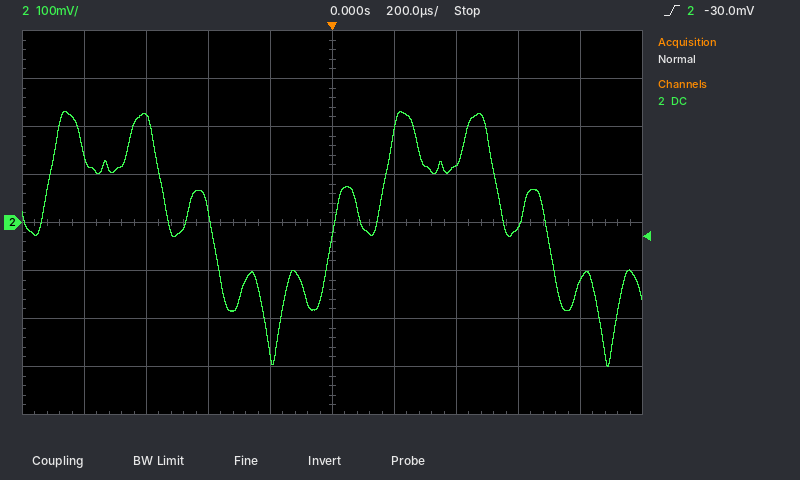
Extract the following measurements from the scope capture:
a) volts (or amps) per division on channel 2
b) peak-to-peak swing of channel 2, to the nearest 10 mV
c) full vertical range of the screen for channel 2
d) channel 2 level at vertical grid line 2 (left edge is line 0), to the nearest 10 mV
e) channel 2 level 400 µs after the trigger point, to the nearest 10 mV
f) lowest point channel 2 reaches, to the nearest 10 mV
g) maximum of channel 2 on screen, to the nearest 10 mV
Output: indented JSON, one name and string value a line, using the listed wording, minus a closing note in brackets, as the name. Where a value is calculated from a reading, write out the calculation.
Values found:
{
  "volts (or amps) per division on channel 2": "100 mV",
  "peak-to-peak swing of channel 2, to the nearest 10 mV": "230 mV − (-300 mV) = 530 mV",
  "full vertical range of the screen for channel 2": "800 mV",
  "channel 2 level at vertical grid line 2 (left edge is line 0), to the nearest 10 mV": "220 mV",
  "channel 2 level 400 µs after the trigger point, to the nearest 10 mV": "120 mV",
  "lowest point channel 2 reaches, to the nearest 10 mV": "-300 mV",
  "maximum of channel 2 on screen, to the nearest 10 mV": "230 mV"
}
